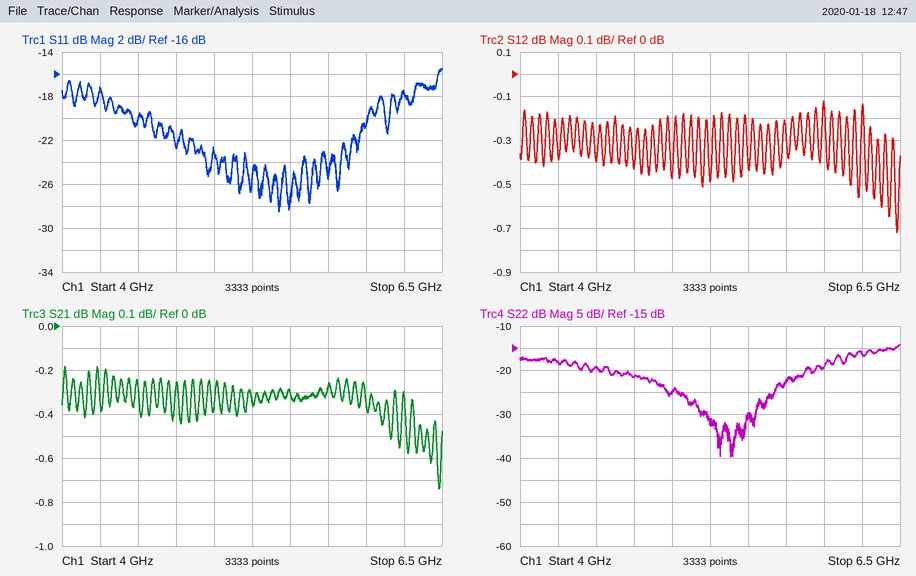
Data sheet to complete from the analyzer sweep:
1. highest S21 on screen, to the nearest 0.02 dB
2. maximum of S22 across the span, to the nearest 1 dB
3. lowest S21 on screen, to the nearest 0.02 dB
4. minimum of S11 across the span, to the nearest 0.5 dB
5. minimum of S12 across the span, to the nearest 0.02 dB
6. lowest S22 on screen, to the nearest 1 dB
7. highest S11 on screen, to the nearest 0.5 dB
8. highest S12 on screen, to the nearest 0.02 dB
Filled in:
-0.18 dB
-14 dB
-0.74 dB
-28.5 dB
-0.72 dB
-40 dB
-15.5 dB
-0.12 dB
